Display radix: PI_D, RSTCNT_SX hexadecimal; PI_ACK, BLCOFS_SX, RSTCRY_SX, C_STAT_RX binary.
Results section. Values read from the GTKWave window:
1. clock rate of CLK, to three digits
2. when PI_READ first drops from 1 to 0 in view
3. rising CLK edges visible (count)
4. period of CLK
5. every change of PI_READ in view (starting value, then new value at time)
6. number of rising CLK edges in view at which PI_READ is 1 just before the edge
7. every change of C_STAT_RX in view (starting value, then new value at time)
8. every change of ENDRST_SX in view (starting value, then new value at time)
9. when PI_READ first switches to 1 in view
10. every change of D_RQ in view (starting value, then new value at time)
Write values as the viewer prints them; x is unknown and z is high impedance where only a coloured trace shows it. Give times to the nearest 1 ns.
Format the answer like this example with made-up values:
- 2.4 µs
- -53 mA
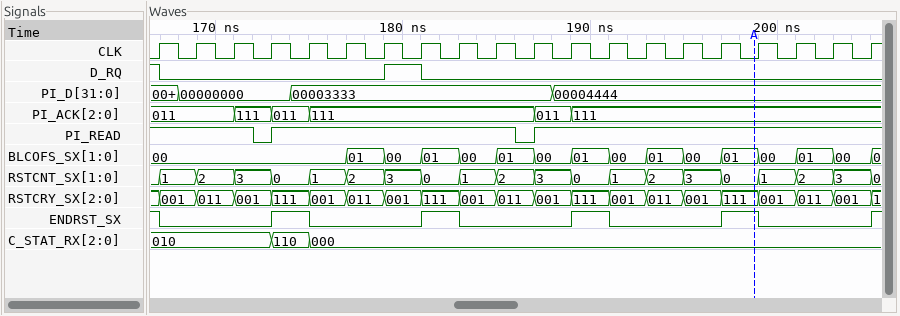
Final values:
- 500 MHz
- 172 ns
- 20
- 2 ns
- 1, 0 at 172 ns, 1 at 173 ns, 0 at 186 ns, 1 at 187 ns
- 18
- 010, 110 at 173 ns, 000 at 175 ns
- 1, 0 at 167 ns, 1 at 173 ns, 0 at 175 ns, 1 at 181 ns, 0 at 183 ns, 1 at 189 ns, 0 at 191 ns, 1 at 197 ns, 0 at 199 ns, 1 at 205 ns
- 173 ns
- 1, 0 at 167 ns, 1 at 179 ns, 0 at 181 ns
